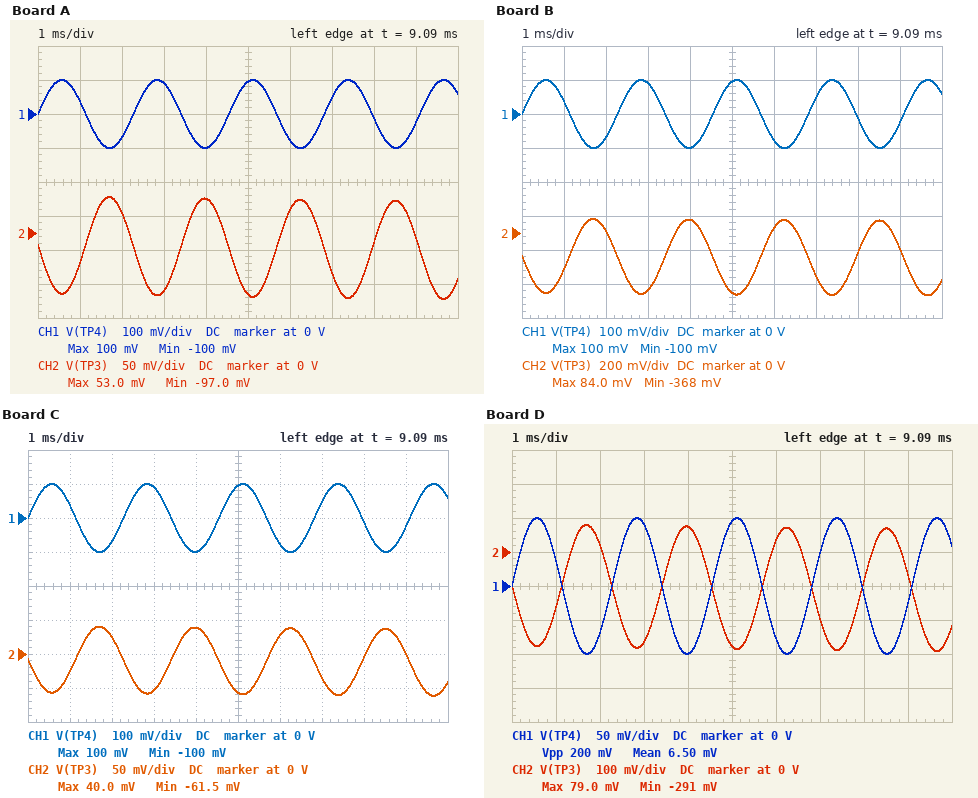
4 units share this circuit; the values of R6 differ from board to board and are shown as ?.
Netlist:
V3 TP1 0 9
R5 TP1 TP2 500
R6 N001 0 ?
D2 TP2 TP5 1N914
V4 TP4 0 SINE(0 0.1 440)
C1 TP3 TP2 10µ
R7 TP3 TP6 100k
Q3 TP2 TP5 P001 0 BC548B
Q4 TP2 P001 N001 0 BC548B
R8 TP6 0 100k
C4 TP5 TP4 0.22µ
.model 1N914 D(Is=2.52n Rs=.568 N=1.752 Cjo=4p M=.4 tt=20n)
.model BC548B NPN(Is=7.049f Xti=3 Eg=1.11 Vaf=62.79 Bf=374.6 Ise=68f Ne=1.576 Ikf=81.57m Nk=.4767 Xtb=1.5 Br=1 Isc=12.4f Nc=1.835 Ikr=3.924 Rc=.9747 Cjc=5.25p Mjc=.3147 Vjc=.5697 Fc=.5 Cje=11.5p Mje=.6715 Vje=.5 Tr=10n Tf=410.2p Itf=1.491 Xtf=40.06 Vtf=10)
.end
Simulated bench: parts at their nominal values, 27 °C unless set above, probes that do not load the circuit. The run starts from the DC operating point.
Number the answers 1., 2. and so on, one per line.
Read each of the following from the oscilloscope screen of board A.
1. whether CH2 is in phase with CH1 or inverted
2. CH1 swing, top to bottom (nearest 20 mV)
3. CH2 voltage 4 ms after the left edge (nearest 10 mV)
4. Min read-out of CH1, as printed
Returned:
1. inverted
2. 200 mV
3. 50 mV
4. -100 mV
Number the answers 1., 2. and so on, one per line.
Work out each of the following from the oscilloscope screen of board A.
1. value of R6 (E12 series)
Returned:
1. 680 Ω
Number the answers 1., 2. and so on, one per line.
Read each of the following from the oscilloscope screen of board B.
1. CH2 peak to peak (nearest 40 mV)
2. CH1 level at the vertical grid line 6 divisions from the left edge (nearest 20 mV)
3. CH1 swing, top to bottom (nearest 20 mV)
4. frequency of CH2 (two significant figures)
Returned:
1. 440 mV
2. -80 mV
3. 200 mV
4. 440 Hz
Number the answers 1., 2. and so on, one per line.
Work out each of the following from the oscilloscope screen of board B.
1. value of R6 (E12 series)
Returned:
1. 220 Ω
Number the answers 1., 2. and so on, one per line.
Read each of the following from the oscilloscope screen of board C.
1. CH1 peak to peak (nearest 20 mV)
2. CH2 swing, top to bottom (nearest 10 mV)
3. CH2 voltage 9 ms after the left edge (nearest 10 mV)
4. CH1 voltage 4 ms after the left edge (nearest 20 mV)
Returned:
1. 200 mV
2. 100 mV
3. 0 V
4. -100 mV
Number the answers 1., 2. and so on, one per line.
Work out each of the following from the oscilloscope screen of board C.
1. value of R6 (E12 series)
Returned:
1. 1 kΩ
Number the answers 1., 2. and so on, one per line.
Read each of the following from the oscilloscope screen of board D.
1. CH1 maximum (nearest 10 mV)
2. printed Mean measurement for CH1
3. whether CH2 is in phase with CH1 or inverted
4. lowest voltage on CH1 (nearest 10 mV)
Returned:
1. 100 mV
2. 6.50 mV
3. inverted
4. -100 mV
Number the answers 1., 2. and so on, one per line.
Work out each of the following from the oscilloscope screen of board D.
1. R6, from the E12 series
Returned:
1. 270 Ω
